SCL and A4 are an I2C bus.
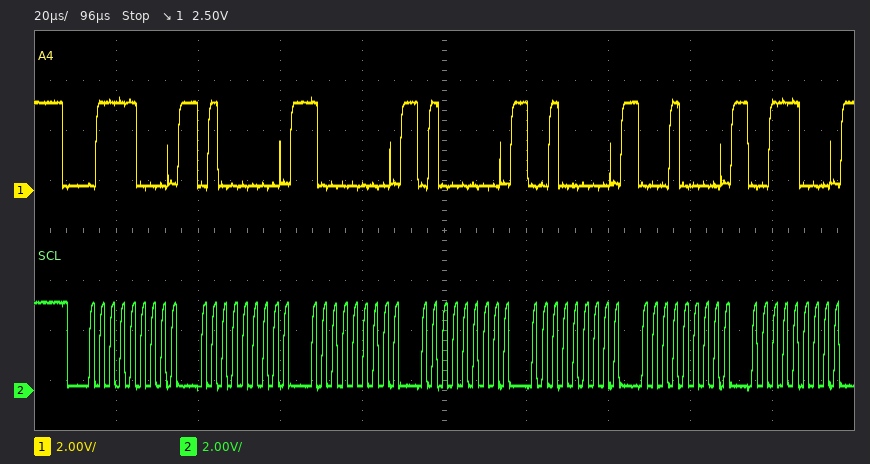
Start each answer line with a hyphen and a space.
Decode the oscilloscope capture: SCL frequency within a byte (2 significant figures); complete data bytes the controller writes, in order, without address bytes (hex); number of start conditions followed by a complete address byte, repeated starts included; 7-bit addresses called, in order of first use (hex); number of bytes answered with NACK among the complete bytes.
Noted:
- 400 kHz
- 40 80 40 20 10 38
- 1
- 0x3C
- 0
